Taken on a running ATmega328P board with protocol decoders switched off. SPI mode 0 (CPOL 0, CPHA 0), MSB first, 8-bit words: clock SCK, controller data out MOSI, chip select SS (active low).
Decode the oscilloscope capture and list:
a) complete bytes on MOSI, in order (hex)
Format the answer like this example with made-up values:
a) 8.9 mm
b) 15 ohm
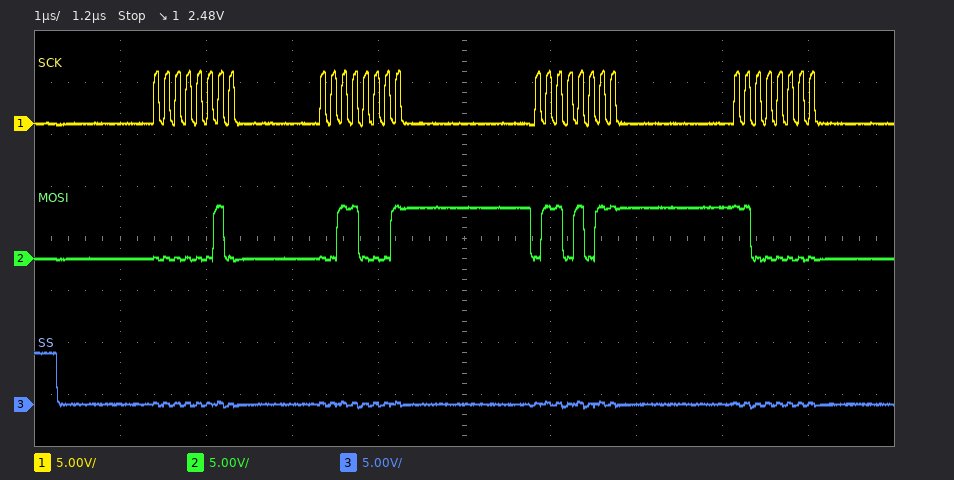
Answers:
a) 0x02 0x31 0x6B 0xC0
